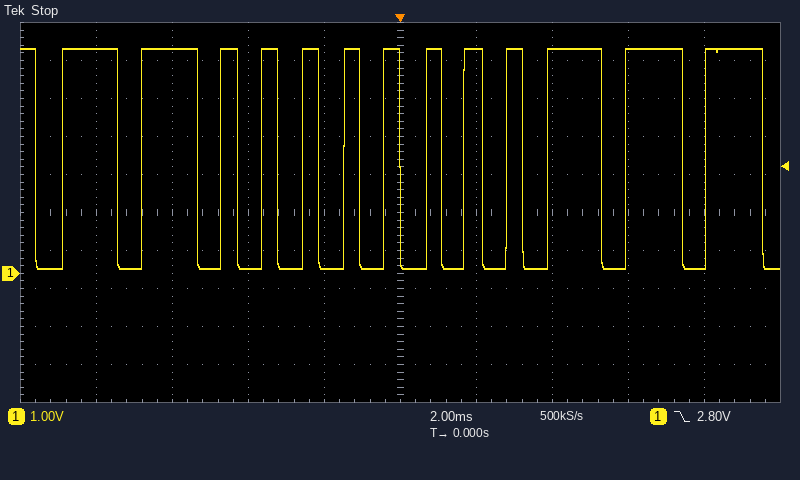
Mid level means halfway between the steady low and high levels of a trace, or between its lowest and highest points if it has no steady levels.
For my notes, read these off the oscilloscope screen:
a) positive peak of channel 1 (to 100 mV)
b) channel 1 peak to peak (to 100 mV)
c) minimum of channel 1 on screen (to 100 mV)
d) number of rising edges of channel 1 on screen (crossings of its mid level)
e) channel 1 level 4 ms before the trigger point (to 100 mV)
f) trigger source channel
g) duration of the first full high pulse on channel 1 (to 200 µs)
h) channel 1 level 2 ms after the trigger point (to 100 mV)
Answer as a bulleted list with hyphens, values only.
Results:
- 5.9 V
- 5.8 V
- 100 mV
- 13
- 100 mV
- channel 1
- 1.4 ms
- 5.9 V
